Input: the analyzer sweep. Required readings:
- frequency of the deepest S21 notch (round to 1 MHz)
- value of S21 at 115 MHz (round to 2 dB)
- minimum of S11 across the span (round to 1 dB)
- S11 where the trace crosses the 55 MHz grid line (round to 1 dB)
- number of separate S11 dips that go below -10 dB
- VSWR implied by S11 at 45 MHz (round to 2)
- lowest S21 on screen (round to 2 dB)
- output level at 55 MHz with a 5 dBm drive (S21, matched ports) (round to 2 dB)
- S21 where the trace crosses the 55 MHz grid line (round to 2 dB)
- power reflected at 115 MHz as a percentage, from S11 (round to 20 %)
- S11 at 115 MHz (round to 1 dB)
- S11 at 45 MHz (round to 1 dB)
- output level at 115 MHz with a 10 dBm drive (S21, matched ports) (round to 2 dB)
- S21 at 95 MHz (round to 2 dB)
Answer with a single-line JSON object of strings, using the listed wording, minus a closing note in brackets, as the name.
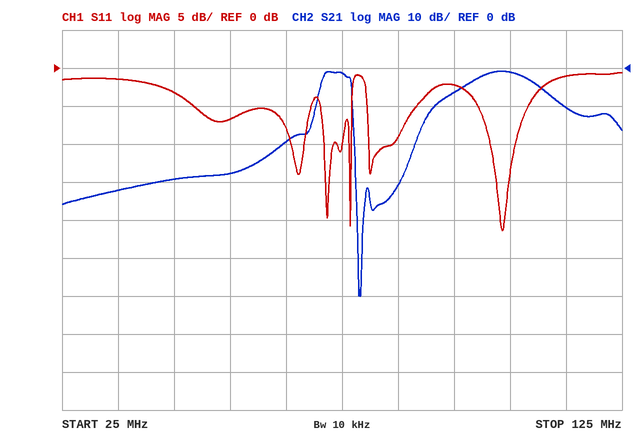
{"frequency of the deepest S21 notch": "78 MHz", "value of S21 at 115 MHz": "-10 dB", "minimum of S11 across the span": "-21 dB", "S11 where the trace crosses the 55 MHz grid line": "-7 dB", "number of separate S11 dips that go below -10 dB": "5", "VSWR implied by S11 at 45 MHz": "6", "lowest S21 on screen": "-60 dB", "output level at 55 MHz with a 5 dBm drive (S21, matched ports)": "-22 dBm", "S21 where the trace crosses the 55 MHz grid line": "-28 dB", "power reflected at 115 MHz as a percentage, from S11": "80 %", "S11 at 115 MHz": "-1 dB", "S11 at 45 MHz": "-3 dB", "output level at 115 MHz with a 10 dBm drive (S21, matched ports)": "0 dBm", "S21 at 95 MHz": "-6 dB"}
